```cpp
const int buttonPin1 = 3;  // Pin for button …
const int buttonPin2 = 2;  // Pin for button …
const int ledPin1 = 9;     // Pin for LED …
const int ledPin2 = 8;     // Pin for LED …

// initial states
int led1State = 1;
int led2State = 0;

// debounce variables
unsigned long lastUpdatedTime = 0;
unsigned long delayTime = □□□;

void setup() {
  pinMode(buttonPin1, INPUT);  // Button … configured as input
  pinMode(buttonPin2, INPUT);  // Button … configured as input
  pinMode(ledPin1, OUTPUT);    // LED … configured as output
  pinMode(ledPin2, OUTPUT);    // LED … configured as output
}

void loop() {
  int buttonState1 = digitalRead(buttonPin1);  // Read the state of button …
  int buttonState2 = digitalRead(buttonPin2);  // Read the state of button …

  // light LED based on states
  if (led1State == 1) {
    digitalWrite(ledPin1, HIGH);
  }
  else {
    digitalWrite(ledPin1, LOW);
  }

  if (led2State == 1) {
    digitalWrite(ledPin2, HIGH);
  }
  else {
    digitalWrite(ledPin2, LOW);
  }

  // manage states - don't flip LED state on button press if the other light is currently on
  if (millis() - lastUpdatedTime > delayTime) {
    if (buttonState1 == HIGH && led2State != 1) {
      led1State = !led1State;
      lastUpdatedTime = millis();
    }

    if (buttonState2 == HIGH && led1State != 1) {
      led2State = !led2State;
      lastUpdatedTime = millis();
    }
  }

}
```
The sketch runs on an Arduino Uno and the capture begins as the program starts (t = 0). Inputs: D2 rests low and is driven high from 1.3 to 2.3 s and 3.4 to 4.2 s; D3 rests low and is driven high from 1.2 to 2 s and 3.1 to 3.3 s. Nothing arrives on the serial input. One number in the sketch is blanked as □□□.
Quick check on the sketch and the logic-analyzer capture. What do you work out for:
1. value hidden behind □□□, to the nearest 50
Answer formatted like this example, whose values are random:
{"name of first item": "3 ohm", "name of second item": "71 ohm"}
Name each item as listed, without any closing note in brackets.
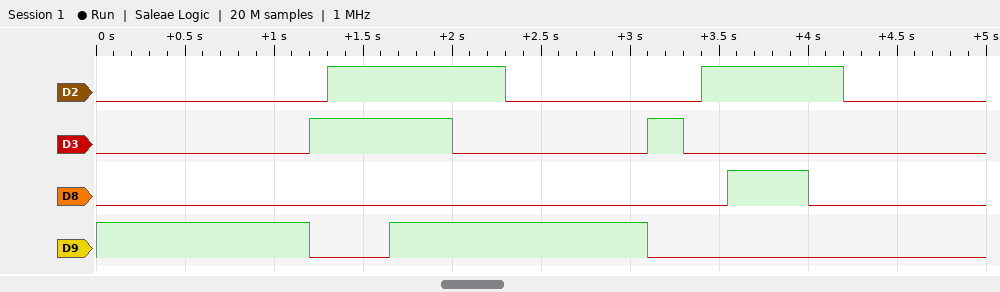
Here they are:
{"value hidden behind □□□, to the nearest 50": "450"}
